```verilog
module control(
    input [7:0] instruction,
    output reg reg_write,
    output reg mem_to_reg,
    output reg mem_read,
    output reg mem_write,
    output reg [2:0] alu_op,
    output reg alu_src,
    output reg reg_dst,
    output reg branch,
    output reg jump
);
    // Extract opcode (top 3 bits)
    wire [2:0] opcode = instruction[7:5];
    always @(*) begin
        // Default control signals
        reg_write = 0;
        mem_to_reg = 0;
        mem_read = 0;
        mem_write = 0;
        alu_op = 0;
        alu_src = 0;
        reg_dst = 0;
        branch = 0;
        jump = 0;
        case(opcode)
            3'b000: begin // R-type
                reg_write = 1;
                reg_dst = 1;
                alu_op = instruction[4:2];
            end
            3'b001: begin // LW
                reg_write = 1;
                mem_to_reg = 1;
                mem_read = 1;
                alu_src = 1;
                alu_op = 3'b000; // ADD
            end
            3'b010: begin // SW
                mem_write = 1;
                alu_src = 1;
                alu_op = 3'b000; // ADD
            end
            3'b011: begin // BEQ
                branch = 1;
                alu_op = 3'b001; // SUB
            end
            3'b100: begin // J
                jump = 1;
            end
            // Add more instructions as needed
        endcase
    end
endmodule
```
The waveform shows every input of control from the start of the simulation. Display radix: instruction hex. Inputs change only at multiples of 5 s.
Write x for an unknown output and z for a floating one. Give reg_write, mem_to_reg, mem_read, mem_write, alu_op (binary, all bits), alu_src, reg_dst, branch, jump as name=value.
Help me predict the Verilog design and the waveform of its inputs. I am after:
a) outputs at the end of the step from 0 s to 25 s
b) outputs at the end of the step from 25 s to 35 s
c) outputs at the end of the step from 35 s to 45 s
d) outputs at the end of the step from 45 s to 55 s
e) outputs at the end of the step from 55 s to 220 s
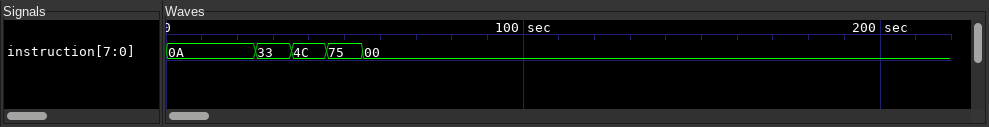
reg_write=1, mem_to_reg=0, mem_read=0, mem_write=0, alu_op=010, alu_src=0, reg_dst=1, branch=0, jump=0
reg_write=1, mem_to_reg=1, mem_read=1, mem_write=0, alu_op=000, alu_src=1, reg_dst=0, branch=0, jump=0
reg_write=0, mem_to_reg=0, mem_read=0, mem_write=1, alu_op=000, alu_src=1, reg_dst=0, branch=0, jump=0
reg_write=0, mem_to_reg=0, mem_read=0, mem_write=0, alu_op=001, alu_src=0, reg_dst=0, branch=1, jump=0
reg_write=1, mem_to_reg=0, mem_read=0, mem_write=0, alu_op=000, alu_src=0, reg_dst=1, branch=0, jump=0
